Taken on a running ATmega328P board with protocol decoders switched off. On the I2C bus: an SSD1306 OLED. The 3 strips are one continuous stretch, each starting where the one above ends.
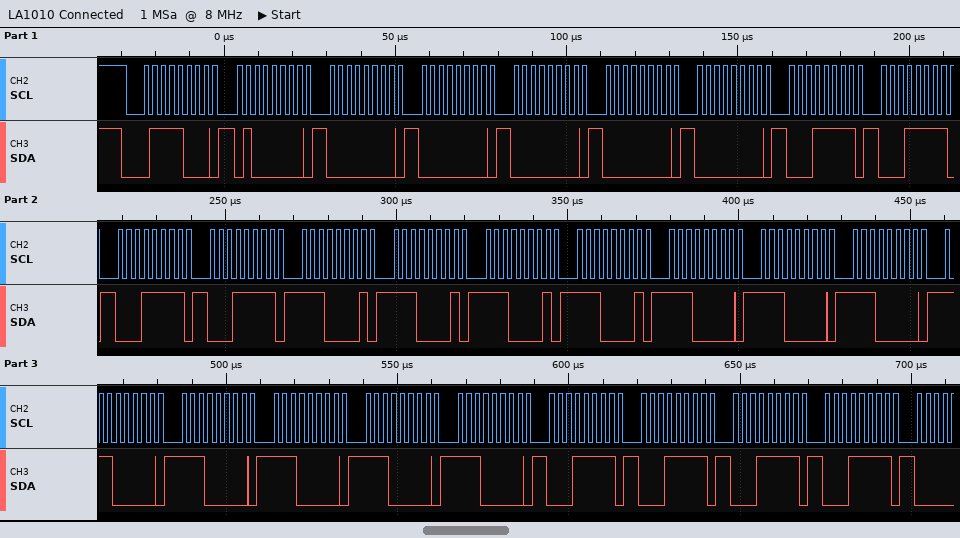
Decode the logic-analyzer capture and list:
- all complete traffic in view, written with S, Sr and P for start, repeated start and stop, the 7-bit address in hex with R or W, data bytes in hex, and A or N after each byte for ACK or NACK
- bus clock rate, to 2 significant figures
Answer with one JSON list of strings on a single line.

["S 3CW A 40 A 00 A 00 A 00 A 00 A 00 A 1F A 1F A 1F A 1F A E1 A E1 A E1 A E1 A E0 A E0 A E0 A E0 A E0 A E0 A E0 A E0 A 1F A 1F A 1F A 1F A", "400 kHz"]
